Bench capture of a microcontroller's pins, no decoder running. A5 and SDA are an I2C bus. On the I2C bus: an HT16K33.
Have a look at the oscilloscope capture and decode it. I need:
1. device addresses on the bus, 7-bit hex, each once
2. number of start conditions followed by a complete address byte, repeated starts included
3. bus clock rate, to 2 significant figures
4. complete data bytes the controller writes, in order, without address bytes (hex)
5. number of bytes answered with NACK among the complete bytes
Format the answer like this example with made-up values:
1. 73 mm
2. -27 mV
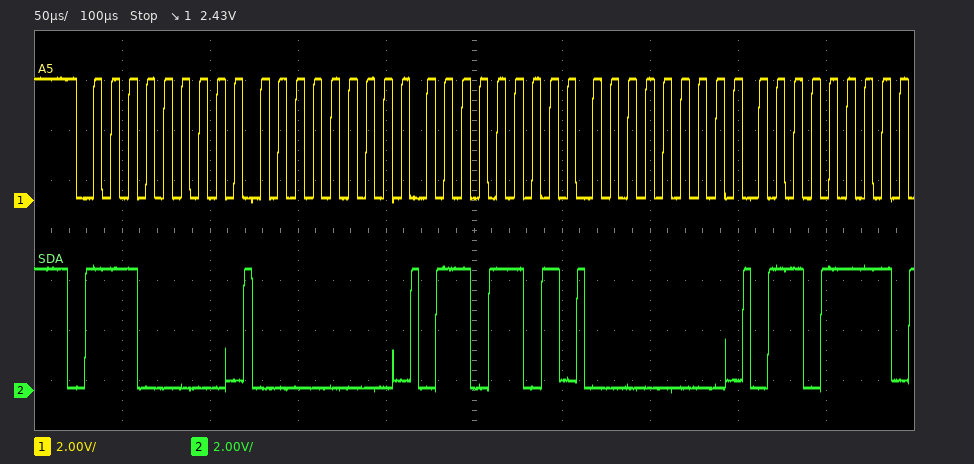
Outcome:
1. 0x70
2. 1
3. 100 kHz
4. 00 6D 00 6F
5. 0
